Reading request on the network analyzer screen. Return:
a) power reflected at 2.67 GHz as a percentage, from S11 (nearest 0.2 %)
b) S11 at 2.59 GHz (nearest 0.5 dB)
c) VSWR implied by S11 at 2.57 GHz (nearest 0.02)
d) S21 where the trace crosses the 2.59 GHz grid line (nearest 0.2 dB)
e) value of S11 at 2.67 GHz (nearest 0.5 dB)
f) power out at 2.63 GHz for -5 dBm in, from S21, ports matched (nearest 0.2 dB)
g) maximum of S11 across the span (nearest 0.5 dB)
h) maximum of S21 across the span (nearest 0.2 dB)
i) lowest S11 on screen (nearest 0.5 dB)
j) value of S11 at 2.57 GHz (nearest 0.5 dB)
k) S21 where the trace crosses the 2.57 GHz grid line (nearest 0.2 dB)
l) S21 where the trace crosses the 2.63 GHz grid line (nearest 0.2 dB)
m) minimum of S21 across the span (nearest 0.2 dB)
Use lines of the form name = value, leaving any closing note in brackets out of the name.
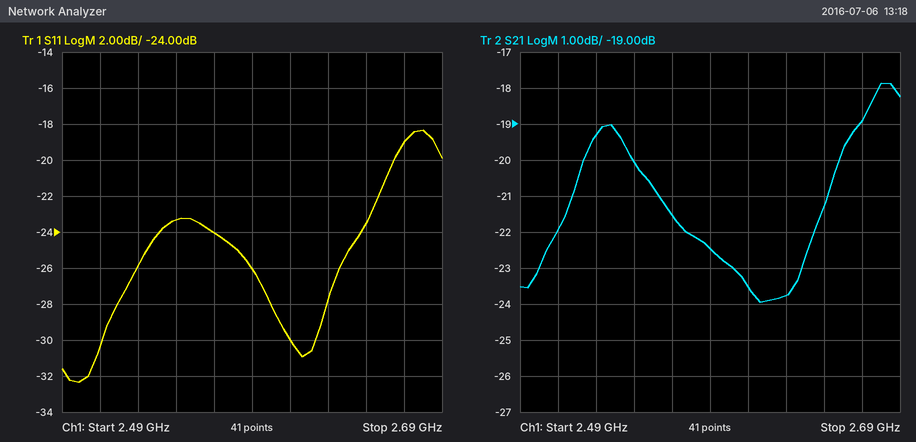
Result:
power reflected at 2.67 GHz as a percentage, from S11 = 1.2 %
S11 at 2.59 GHz = -26.0 dB
VSWR implied by S11 at 2.57 GHz = 1.14
S21 where the trace crosses the 2.59 GHz grid line = -22.4 dB
value of S11 at 2.67 GHz = -19.0 dB
power out at 2.63 GHz for -5 dBm in, from S21, ports matched = -28.8 dBm
maximum of S11 across the span = -18.5 dB
maximum of S21 across the span = -17.8 dB
lowest S11 on screen = -32.5 dB
value of S11 at 2.57 GHz = -24.0 dB
S21 where the trace crosses the 2.57 GHz grid line = -21.6 dB
S21 where the trace crosses the 2.63 GHz grid line = -23.8 dB
minimum of S21 across the span = -24.0 dB
